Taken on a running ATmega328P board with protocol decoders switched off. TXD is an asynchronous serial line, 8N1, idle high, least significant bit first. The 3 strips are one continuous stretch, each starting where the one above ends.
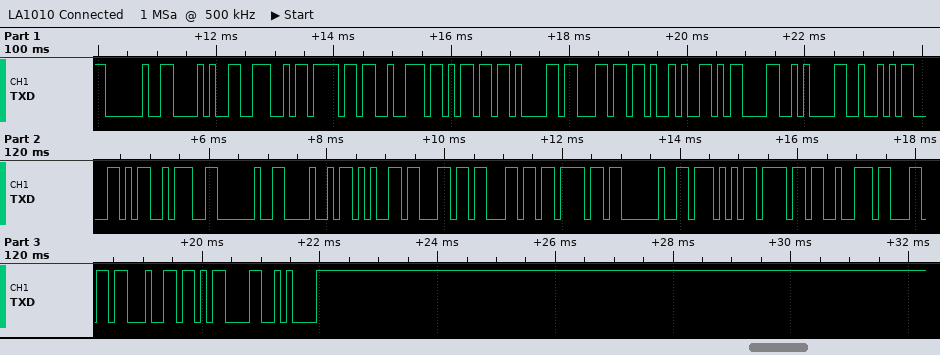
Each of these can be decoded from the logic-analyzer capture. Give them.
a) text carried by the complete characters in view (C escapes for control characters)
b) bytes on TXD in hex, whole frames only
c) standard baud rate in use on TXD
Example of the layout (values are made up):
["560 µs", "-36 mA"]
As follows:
["\" (Normal)\\r\\nRX: Hello World\\r\\n\"", "0x20 0x28 0x4E 0x6F 0x72 0x6D 0x61 0x6C 0x29 0x0D 0x0A 0x52 0x58 0x3A 0x20 0x48 0x65 0x6C 0x6C 0x6F 0x20 0x57 0x6F 0x72 0x6C 0x64 0x0D 0x0A", "9600 baud"]
